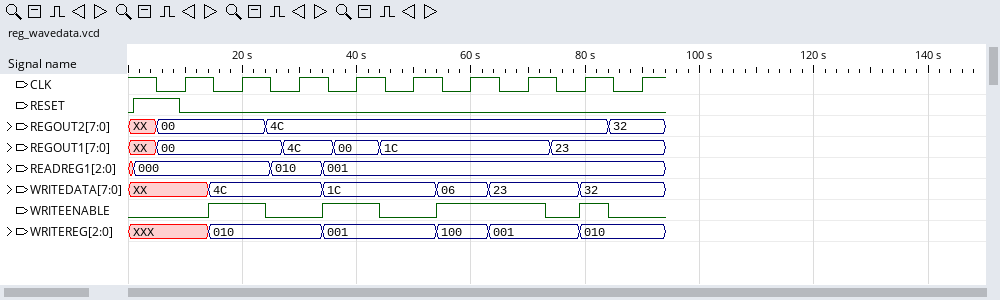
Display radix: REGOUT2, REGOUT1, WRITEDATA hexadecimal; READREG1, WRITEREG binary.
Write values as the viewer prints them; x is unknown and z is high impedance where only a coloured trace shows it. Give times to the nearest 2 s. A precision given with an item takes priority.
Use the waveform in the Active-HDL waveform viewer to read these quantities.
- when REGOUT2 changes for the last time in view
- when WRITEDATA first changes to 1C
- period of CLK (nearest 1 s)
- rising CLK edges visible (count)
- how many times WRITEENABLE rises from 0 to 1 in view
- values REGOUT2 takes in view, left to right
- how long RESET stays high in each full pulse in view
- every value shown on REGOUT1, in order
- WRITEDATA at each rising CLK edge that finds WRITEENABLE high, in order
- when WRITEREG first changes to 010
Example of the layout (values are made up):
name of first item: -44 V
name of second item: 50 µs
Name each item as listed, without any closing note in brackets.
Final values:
when REGOUT2 changes for the last time in view: 84 s
when WRITEDATA first changes to 1C: 34 s
period of CLK: 10 s
rising CLK edges visible: 9
how many times WRITEENABLE rises from 0 to 1 in view: 4
values REGOUT2 takes in view, left to right: XX, 00, 4C, 32
how long RESET stays high in each full pulse in view: 8 s
every value shown on REGOUT1, in order: XX, 00, 4C, 00, 1C, 23
WRITEDATA at each rising CLK edge that finds WRITEENABLE high, in order: 4C, 1C, 06, 23, 32
when WRITEREG first changes to 010: 14 s
